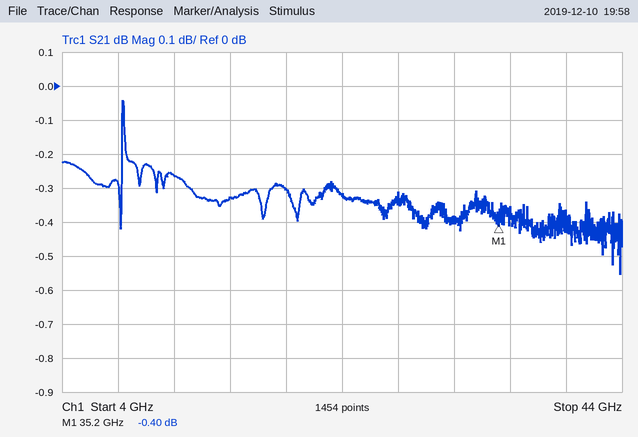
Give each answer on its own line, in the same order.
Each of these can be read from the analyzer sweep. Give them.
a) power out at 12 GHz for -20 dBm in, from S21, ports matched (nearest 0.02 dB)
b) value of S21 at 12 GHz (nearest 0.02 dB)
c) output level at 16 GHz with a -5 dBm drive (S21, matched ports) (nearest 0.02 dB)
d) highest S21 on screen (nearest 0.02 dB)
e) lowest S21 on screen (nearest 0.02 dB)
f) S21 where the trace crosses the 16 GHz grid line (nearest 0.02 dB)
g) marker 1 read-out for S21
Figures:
-20.26 dBm
-0.26 dB
-5.32 dBm
-0.04 dB
-0.56 dB
-0.32 dB
-0.40 dB
